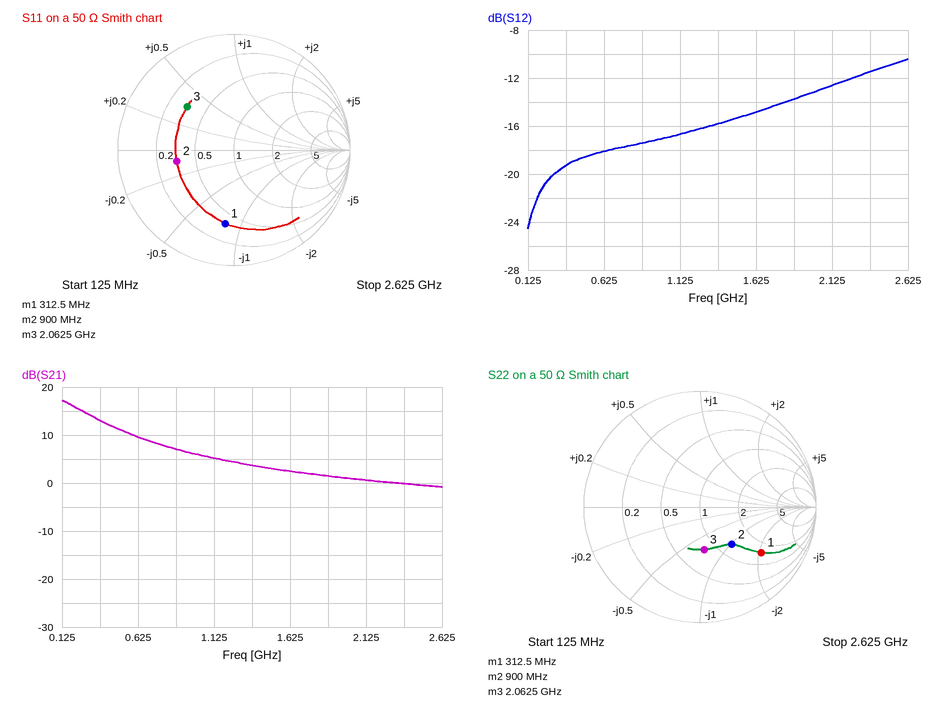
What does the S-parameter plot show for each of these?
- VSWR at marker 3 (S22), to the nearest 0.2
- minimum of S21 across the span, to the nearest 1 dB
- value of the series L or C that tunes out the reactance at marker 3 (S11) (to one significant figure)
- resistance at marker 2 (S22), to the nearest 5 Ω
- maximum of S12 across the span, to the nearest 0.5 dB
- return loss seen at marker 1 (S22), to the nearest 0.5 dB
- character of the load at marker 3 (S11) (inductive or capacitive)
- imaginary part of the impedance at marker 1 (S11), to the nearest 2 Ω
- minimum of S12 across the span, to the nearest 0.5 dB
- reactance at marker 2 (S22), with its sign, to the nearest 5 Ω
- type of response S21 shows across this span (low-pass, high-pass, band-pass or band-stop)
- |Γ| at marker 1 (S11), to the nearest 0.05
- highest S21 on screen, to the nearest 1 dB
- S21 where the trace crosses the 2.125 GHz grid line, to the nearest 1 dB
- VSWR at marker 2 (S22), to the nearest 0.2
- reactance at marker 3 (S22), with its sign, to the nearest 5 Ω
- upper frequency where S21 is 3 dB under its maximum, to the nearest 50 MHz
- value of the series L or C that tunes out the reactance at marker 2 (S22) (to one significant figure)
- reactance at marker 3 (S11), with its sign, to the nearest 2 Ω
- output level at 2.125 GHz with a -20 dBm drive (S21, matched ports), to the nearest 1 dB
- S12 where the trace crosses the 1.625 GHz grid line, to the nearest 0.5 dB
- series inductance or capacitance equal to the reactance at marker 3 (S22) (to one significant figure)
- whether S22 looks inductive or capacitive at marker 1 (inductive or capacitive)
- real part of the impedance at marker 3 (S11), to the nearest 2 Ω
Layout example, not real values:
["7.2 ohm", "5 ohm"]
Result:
["2.2", "-1 dB", "4 pF", "65 Ω", "-10.5 dB", "3.5 dB", "inductive", "-40 Ω", "-24.5 dB", "-50 Ω", "low-pass", "0.65", "17 dB", "1 dB", "2.4", "-35 Ω", "300 MHz", "9 nH", "+18 Ω", "-19 dBm", "-15.0 dB", "2 pF", "capacitive", "16 Ω"]
